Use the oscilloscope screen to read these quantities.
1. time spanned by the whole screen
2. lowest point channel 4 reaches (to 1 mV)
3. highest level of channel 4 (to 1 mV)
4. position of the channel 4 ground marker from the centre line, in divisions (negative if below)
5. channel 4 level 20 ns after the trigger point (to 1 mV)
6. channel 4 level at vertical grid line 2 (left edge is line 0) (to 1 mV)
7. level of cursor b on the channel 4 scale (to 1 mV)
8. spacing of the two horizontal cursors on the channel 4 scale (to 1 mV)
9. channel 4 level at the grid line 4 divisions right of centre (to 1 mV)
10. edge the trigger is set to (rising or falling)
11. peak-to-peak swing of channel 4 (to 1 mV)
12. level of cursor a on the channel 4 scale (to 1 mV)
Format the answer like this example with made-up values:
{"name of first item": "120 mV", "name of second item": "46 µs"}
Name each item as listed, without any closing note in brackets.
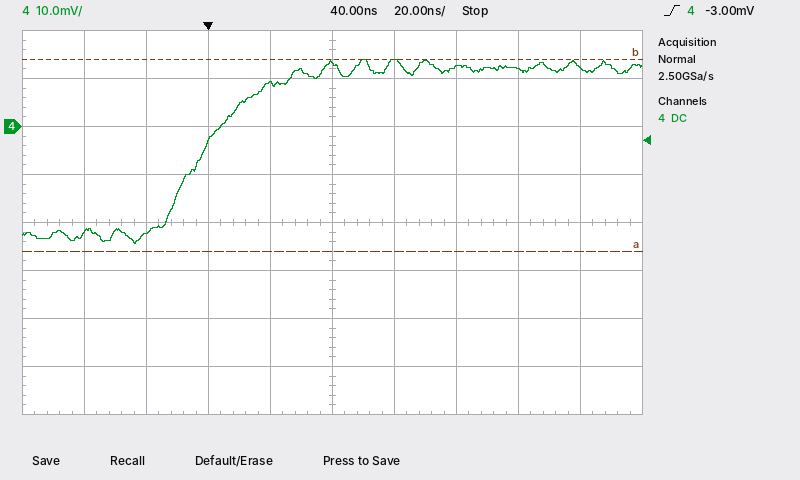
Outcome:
{"time spanned by the whole screen": "200 ns", "lowest point channel 4 reaches": "-24 mV", "highest level of channel 4": "14 mV", "position of the channel 4 ground marker from the centre line, in divisions": "+2.0 div", "channel 4 level 20 ns after the trigger point": "9 mV", "channel 4 level at vertical grid line 2 (left edge is line 0)": "-22 mV", "level of cursor b on the channel 4 scale": "14 mV", "spacing of the two horizontal cursors on the channel 4 scale": "40 mV", "channel 4 level at the grid line 4 divisions right of centre": "12 mV", "edge the trigger is set to": "rising", "peak-to-peak swing of channel 4": "38 mV", "level of cursor a on the channel 4 scale": "-26 mV"}
